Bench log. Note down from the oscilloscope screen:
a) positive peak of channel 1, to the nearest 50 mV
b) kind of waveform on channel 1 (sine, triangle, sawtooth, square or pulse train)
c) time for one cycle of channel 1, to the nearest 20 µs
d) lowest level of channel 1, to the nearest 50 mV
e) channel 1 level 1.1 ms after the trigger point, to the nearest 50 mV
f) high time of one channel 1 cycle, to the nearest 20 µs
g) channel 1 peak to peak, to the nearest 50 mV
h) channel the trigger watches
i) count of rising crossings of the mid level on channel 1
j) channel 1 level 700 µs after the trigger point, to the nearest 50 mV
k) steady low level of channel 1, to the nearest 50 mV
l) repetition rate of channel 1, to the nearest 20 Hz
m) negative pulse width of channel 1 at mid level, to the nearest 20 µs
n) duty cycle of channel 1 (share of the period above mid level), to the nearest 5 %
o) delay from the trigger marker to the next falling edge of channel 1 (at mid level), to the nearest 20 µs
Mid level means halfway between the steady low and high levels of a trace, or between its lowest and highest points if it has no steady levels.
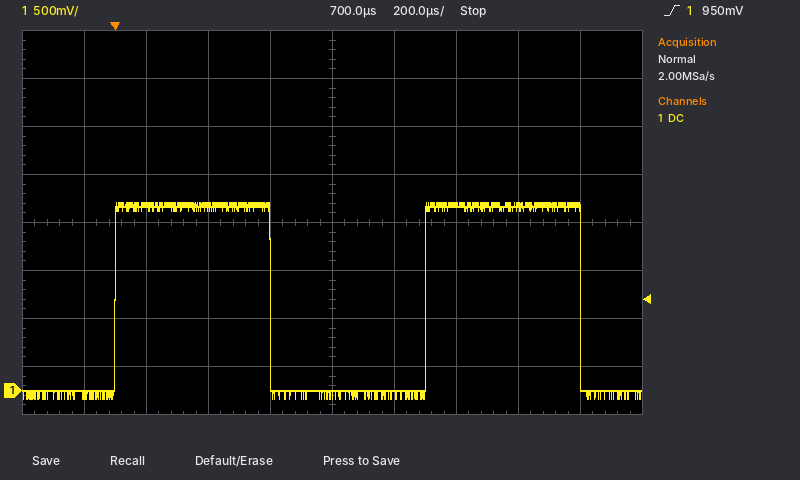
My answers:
1.95 V
square
1.00 ms
-100 mV
1.95 V
500 µs
2.05 V
channel 1
2
-50 mV
0 mV
1.00 kHz
500 µs
50 %
500 µs
